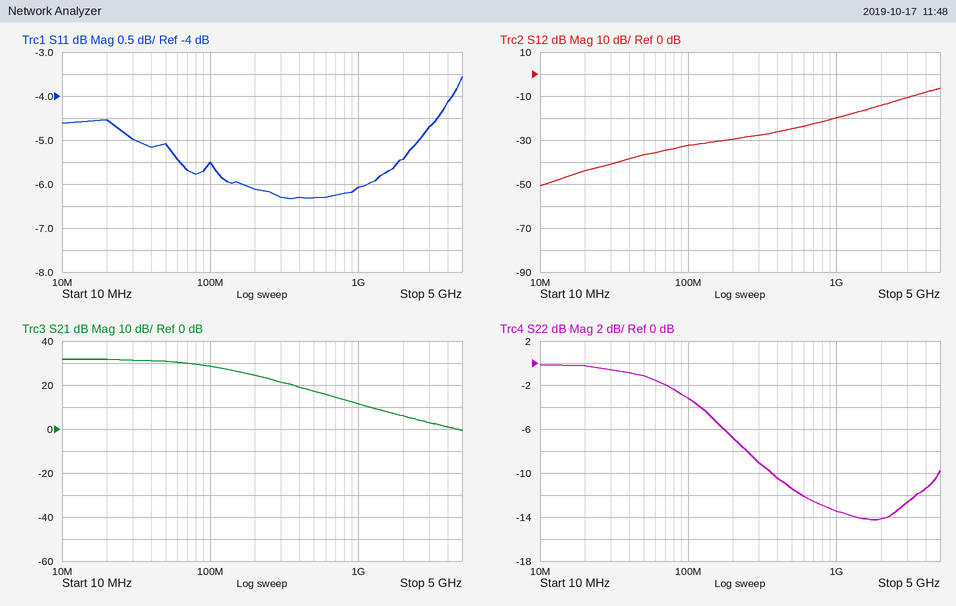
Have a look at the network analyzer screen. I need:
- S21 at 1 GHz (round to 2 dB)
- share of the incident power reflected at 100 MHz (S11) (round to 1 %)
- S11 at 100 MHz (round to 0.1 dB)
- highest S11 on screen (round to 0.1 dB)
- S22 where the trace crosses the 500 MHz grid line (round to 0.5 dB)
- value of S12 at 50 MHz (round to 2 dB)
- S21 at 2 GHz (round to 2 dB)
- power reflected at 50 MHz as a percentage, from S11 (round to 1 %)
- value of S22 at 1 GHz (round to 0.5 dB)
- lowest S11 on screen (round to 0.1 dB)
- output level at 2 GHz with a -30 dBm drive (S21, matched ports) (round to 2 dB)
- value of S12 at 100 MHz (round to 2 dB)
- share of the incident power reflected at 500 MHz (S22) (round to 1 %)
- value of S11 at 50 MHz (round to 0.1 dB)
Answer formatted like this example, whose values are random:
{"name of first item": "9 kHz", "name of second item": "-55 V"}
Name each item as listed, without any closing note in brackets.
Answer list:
{"S21 at 1 GHz": "12 dB", "share of the incident power reflected at 100 MHz (S11)": "28 %", "S11 at 100 MHz": "-5.5 dB", "highest S11 on screen": "-3.6 dB", "S22 where the trace crosses the 500 MHz grid line": "-11.5 dB", "value of S12 at 50 MHz": "-36 dB", "S21 at 2 GHz": "6 dB", "power reflected at 50 MHz as a percentage, from S11": "31 %", "value of S22 at 1 GHz": "-13.5 dB", "lowest S11 on screen": "-6.3 dB", "output level at 2 GHz with a -30 dBm drive (S21, matched ports)": "-24 dBm", "value of S12 at 100 MHz": "-32 dB", "share of the incident power reflected at 500 MHz (S22)": "7 %", "value of S11 at 50 MHz": "-5.1 dB"}
